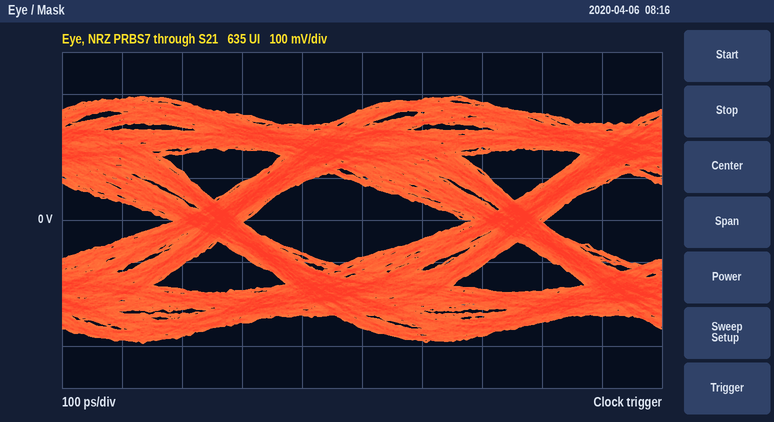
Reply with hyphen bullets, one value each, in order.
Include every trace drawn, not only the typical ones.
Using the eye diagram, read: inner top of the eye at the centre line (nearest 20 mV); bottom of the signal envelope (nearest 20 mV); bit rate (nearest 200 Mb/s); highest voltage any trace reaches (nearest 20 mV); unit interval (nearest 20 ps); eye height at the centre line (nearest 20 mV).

- 80 mV
- -300 mV
- 2.0 Gb/s
- 300 mV
- 500 ps
- 180 mV
